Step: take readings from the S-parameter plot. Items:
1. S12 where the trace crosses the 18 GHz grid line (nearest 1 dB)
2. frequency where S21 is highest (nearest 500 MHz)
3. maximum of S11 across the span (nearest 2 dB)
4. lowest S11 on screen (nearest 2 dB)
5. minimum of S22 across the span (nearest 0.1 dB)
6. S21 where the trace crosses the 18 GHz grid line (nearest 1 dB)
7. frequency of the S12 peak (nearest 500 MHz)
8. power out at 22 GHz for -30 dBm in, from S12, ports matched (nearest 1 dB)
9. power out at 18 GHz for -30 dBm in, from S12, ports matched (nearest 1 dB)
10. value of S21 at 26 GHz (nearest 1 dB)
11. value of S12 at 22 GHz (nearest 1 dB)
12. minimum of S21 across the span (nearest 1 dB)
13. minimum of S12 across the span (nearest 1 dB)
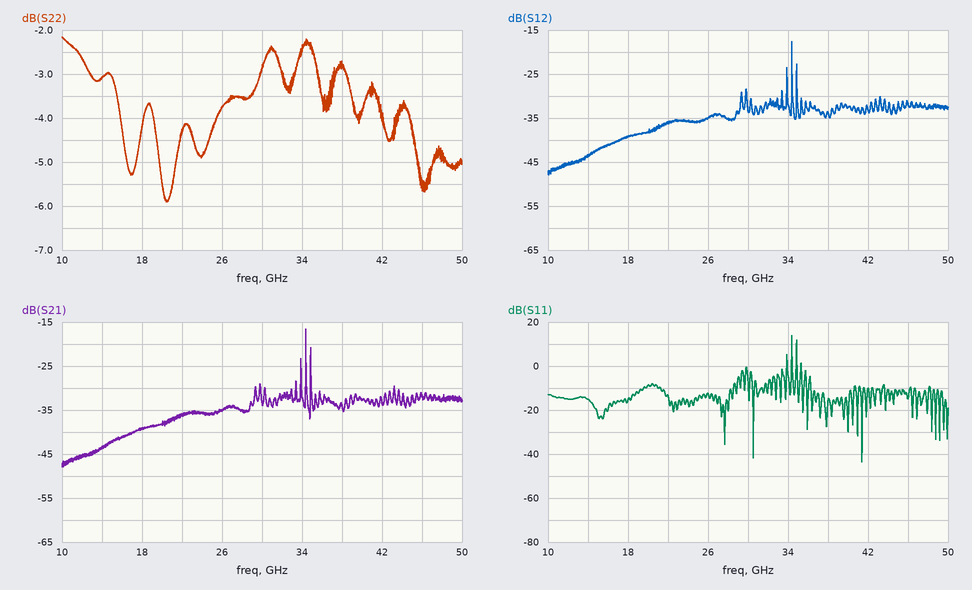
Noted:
-39 dB
34.5 GHz
14 dB
-44 dB
-5.9 dB
-39 dB
34.5 GHz
-66 dBm
-69 dBm
-35 dB
-36 dB
-48 dB
-48 dB
